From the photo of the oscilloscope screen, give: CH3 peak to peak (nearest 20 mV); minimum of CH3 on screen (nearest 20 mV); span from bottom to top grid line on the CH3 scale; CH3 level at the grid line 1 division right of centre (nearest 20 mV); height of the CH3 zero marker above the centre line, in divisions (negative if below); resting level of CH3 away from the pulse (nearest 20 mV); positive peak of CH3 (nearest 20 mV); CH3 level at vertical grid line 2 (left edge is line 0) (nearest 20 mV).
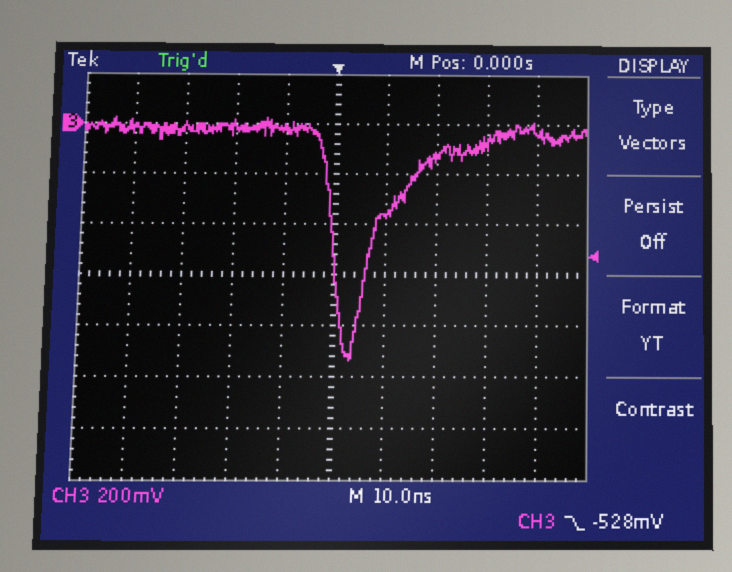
960 mV
-940 mV
1.6 V
-360 mV
+3.0 div
-20 mV
20 mV
-20 mV
